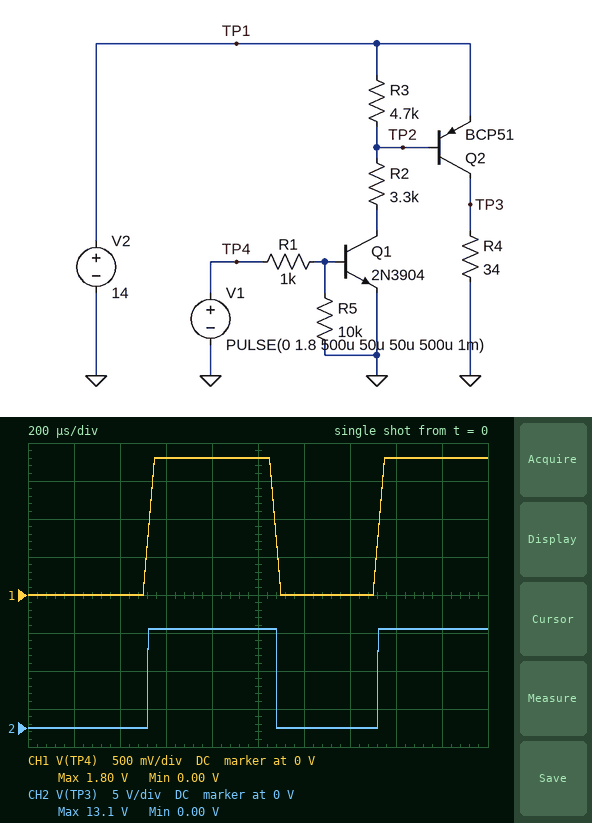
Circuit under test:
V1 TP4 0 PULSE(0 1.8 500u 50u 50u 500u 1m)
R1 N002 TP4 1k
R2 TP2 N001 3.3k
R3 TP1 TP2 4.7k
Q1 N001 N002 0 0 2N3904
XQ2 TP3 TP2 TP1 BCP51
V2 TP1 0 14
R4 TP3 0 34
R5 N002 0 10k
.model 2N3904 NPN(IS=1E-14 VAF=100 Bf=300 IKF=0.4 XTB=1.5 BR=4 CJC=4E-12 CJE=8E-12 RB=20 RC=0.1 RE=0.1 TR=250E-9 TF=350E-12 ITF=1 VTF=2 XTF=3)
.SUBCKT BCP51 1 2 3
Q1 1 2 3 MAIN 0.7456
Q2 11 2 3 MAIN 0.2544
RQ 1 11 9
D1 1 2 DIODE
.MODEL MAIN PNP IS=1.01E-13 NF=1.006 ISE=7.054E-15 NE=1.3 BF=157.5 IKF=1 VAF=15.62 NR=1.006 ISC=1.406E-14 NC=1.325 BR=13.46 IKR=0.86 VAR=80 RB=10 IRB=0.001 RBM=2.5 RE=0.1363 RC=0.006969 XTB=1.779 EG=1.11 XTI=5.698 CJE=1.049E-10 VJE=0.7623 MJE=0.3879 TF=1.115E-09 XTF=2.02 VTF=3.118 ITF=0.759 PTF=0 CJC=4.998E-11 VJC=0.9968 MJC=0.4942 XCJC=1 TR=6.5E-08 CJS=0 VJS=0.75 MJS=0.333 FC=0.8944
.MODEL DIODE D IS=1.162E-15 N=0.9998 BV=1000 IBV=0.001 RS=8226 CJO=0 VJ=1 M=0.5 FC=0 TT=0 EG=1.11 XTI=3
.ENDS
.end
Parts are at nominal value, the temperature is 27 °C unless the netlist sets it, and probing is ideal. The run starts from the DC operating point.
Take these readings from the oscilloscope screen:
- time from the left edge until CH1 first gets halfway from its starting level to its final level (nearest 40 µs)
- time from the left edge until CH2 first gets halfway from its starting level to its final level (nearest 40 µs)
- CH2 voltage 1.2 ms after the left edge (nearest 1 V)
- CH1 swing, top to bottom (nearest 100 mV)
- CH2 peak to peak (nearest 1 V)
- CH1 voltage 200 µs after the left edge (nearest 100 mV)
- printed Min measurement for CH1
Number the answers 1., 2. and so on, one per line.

1. 520 µs
2. 520 µs
3. 0 V
4. 1.8 V
5. 13 V
6. 0 V
7. 0.00 V
